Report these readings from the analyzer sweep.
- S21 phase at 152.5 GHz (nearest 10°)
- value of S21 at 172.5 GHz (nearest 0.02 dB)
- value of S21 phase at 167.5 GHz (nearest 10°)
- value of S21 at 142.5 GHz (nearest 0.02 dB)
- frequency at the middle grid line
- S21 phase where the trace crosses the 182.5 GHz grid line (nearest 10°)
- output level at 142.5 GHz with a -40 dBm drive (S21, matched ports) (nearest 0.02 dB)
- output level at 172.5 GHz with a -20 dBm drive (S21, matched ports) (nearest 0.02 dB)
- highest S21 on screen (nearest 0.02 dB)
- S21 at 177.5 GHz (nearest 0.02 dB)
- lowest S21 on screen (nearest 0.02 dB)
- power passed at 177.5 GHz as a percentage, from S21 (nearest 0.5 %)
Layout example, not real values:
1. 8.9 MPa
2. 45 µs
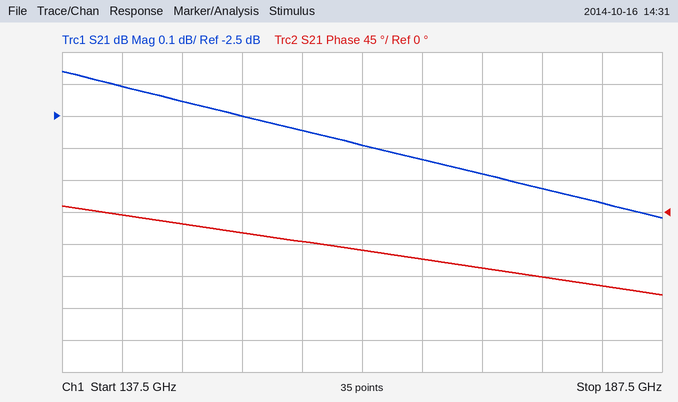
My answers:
1. -30°
2. -2.68 dB
3. -70°
4. -2.40 dB
5. 162.5 GHz
6. -100°
7. -42.40 dBm
8. -22.68 dBm
9. -2.36 dB
10. -2.72 dB
11. -2.82 dB
12. 53.5 %
